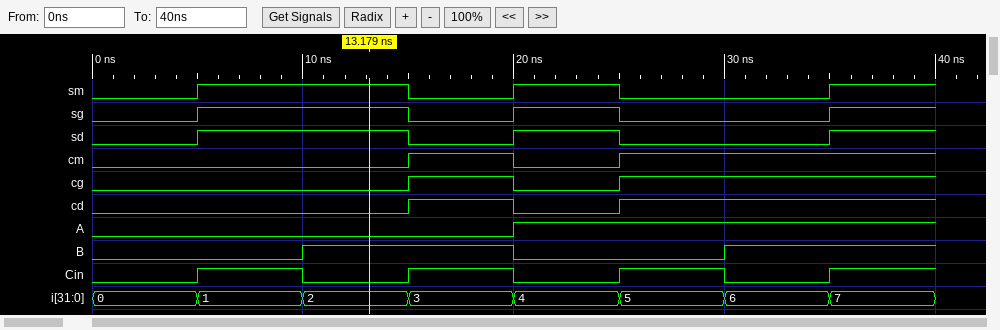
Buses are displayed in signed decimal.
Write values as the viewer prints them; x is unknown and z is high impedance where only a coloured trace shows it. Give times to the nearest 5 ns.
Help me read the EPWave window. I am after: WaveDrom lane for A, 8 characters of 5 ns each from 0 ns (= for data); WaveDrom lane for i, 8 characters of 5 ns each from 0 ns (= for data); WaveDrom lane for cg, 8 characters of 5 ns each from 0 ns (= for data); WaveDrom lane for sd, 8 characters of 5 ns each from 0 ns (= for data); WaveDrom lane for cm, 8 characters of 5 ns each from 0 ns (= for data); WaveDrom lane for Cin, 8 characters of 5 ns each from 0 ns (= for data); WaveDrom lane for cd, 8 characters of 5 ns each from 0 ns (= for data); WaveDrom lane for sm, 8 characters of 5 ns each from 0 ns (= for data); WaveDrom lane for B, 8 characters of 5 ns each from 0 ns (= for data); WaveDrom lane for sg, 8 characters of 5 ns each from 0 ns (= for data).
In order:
{name: 'A', wave: '0...1...'}
{name: 'i', wave: '========', data: '0 1 2 3 4 5 6 7'}
{name: 'cg', wave: '0..101..'}
{name: 'sd', wave: '01.010.1'}
{name: 'cm', wave: '0..101..'}
{name: 'Cin', wave: '01010101'}
{name: 'cd', wave: '0..101..'}
{name: 'sm', wave: '01.010.1'}
{name: 'B', wave: '0.1.0.1.'}
{name: 'sg', wave: '01.010.1'}
